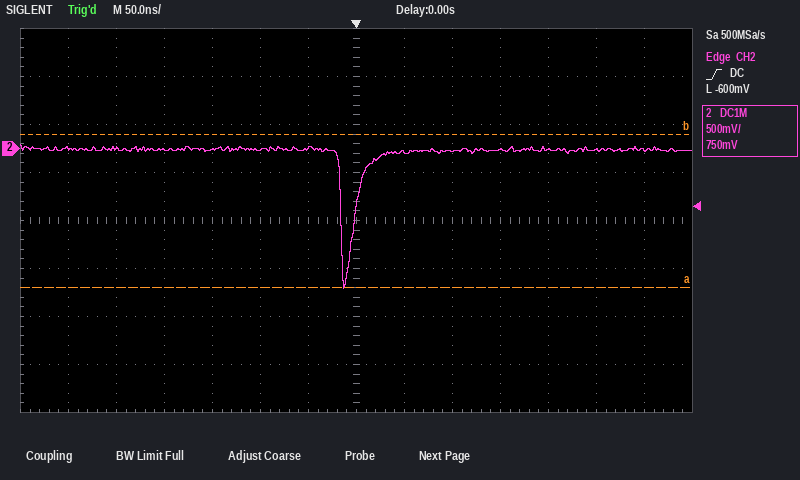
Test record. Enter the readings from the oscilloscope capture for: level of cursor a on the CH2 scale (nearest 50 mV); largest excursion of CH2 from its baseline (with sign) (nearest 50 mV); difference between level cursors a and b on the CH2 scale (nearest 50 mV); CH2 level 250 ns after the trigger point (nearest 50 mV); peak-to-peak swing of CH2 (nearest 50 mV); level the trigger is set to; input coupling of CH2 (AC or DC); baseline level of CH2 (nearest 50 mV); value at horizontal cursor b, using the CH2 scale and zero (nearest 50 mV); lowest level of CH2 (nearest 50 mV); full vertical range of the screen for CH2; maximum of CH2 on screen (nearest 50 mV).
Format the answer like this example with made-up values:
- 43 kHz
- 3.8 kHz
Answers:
- -1.45 V
- -1.45 V
- 1.60 V
- 0 mV
- 1.50 V
- -600 mV
- DC
- 0 mV
- 150 mV
- -1.45 V
- 4 V
- 50 mV
